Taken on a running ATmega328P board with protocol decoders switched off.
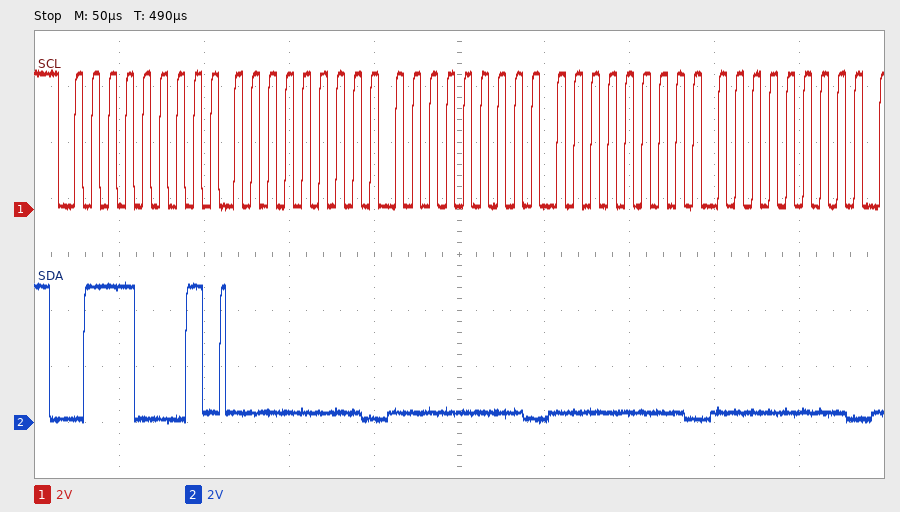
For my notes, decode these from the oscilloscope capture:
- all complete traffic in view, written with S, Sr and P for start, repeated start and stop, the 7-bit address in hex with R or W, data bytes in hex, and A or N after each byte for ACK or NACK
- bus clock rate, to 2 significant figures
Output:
S 38R A 00 A 00 A 00 A 00 A
100 kHz
